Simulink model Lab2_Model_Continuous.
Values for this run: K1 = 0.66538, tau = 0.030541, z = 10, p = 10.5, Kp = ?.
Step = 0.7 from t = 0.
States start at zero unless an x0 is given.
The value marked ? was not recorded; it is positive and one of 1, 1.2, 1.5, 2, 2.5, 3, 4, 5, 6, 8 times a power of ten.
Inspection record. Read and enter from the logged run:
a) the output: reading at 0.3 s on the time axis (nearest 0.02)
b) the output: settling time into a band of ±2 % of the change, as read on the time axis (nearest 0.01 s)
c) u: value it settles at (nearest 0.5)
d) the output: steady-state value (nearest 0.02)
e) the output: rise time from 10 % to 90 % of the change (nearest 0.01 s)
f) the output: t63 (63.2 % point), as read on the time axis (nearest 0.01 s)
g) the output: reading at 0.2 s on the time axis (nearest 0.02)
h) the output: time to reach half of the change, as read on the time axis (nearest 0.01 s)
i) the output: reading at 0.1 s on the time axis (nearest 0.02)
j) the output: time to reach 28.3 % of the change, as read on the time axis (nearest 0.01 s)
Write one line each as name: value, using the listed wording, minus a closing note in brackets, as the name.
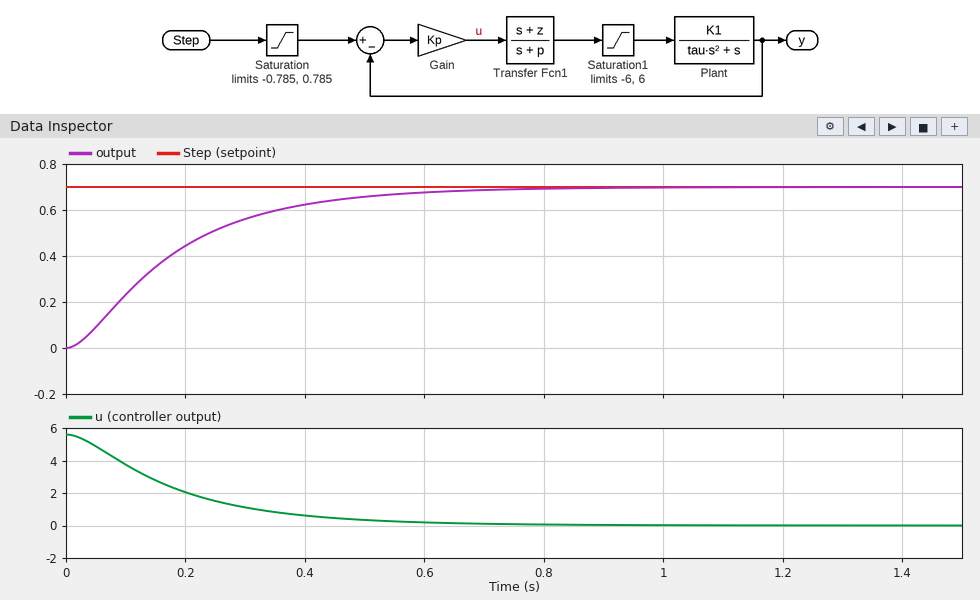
the output: reading at 0.3 s on the time axis: 0.56
the output: settling time into a band of ±2 % of the change, as read on the time axis: 0.69 s
u: value it settles at: 0.0
the output: steady-state value: 0.70
the output: rise time from 10 % to 90 % of the change: 0.37 s
the output: t63 (63.2 % point), as read on the time axis: 0.20 s
the output: reading at 0.2 s on the time axis: 0.44
the output: time to reach half of the change, as read on the time axis: 0.15 s
the output: reading at 0.1 s on the time axis: 0.24
the output: time to reach 28.3 % of the change, as read on the time axis: 0.09 s
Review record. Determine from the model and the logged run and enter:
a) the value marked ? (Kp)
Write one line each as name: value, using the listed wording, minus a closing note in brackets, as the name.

the value marked ?: 8
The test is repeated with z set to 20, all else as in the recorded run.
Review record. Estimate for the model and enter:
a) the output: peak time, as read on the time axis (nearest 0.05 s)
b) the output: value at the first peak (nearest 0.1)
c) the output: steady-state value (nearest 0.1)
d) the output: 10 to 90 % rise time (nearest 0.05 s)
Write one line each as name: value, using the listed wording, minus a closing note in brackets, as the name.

the output: peak time, as read on the time axis: 0.35 s
the output: value at the first peak: 0.8
the output: steady-state value: 0.7
the output: 10 to 90 % rise time: 0.15 s
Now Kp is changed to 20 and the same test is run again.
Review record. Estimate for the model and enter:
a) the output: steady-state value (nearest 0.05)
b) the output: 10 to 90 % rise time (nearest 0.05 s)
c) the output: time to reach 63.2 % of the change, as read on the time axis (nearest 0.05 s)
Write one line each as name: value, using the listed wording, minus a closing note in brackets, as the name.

the output: steady-state value: 0.70
the output: 10 to 90 % rise time: 0.15 s
the output: time to reach 63.2 % of the change, as read on the time axis: 0.15 s
